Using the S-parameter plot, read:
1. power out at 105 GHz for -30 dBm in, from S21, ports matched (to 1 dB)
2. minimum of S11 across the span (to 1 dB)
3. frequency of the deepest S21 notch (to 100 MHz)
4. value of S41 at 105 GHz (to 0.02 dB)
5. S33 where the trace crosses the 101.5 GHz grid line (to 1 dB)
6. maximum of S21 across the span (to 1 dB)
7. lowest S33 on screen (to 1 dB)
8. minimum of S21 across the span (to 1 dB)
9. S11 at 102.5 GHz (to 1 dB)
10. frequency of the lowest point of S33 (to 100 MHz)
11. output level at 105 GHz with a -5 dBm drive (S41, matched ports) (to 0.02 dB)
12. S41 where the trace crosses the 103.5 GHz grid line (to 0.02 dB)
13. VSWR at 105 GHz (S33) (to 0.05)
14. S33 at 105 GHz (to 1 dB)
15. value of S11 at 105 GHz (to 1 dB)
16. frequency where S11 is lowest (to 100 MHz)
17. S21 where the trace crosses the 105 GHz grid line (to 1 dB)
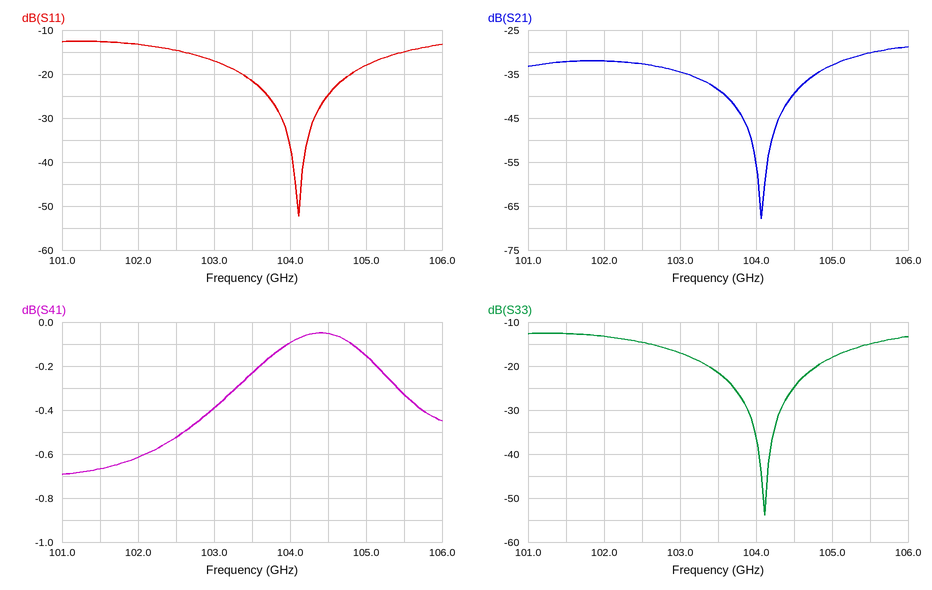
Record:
-63 dBm
-52 dB
104.1 GHz
-0.16 dB
-13 dB
-29 dB
-54 dB
-68 dB
-15 dB
104.1 GHz
-5.16 dBm
-0.24 dB
1.30
-18 dB
-18 dB
104.1 GHz
-33 dB
